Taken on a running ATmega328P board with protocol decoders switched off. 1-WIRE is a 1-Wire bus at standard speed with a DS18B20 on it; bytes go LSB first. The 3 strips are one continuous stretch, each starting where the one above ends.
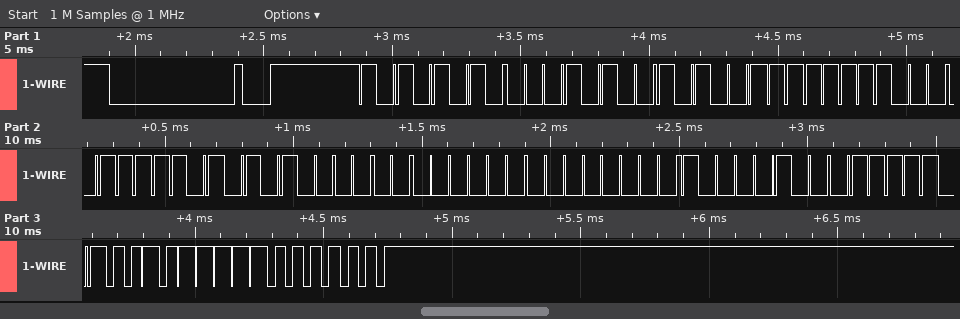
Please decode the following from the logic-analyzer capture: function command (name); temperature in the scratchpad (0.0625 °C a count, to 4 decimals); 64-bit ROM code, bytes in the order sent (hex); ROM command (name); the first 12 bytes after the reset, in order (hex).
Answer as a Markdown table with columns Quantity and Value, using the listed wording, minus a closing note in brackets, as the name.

| Quantity | Value |
|---|---|
| function command | Read Scratchpad |
| temperature in the scratchpad | 31.2500 °C |
| 64-bit ROM code, bytes in the order sent | 28 E5 1F BE 0A 00 00 21 |
| ROM command | Match ROM |
| the first 12 bytes after the reset, in order | 55 28 E5 1F BE 0A 00 00 21 BE F4 01 |
